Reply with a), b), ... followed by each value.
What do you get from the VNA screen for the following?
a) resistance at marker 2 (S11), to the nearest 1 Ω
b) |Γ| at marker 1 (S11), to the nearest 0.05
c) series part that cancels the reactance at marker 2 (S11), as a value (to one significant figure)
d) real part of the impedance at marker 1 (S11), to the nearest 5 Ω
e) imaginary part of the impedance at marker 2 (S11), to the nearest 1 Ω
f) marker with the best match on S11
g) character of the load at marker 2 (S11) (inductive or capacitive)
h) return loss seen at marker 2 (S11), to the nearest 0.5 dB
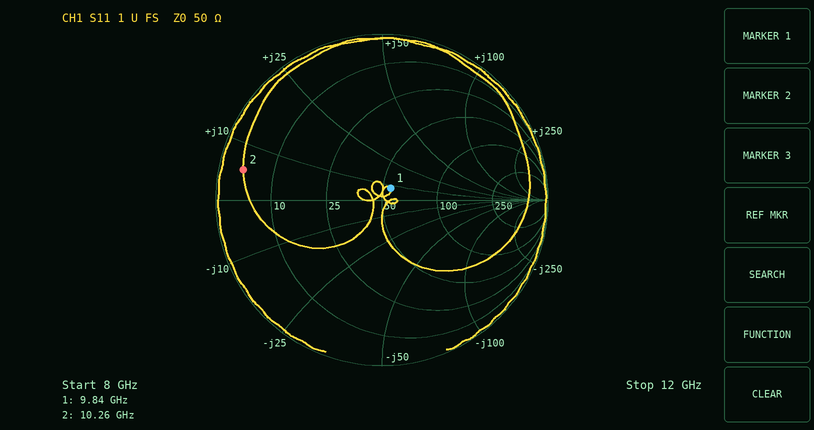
a) 4 Ω
b) 0.10
c) 3 pF
d) 55 Ω
e) +5 Ω
f) marker 1
g) inductive
h) 1.5 dB
